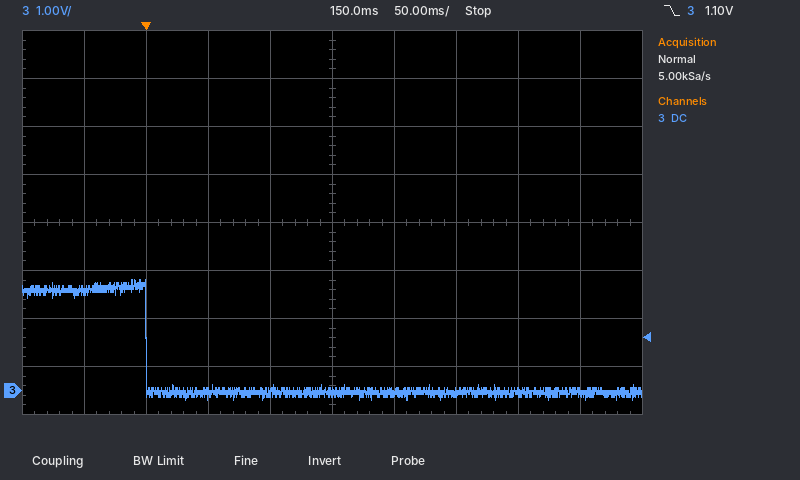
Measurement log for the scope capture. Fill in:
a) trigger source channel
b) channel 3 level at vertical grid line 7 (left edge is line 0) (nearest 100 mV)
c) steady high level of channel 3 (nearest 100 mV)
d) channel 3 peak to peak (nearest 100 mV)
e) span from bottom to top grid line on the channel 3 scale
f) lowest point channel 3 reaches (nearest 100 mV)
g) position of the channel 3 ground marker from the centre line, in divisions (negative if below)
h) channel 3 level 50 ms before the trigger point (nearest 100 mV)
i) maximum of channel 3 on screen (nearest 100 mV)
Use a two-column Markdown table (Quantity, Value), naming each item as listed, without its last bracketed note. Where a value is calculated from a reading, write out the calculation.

| Quantity | Value |
|---|---|
| trigger source channel | channel 3 |
| channel 3 level at vertical grid line 7 (left edge is line 0) | 0.0 V |
| steady high level of channel 3 | 2.1 V |
| channel 3 peak to peak | 2.3 V − (-200 mV) = 2.5 V |
| span from bottom to top grid line on the channel 3 scale | 8 V |
| lowest point channel 3 reaches | -200 mV |
| position of the channel 3 ground marker from the centre line, in divisions | -3.5 div |
| channel 3 level 50 ms before the trigger point | 2.1 V |
| maximum of channel 3 on screen | 2.3 V |
